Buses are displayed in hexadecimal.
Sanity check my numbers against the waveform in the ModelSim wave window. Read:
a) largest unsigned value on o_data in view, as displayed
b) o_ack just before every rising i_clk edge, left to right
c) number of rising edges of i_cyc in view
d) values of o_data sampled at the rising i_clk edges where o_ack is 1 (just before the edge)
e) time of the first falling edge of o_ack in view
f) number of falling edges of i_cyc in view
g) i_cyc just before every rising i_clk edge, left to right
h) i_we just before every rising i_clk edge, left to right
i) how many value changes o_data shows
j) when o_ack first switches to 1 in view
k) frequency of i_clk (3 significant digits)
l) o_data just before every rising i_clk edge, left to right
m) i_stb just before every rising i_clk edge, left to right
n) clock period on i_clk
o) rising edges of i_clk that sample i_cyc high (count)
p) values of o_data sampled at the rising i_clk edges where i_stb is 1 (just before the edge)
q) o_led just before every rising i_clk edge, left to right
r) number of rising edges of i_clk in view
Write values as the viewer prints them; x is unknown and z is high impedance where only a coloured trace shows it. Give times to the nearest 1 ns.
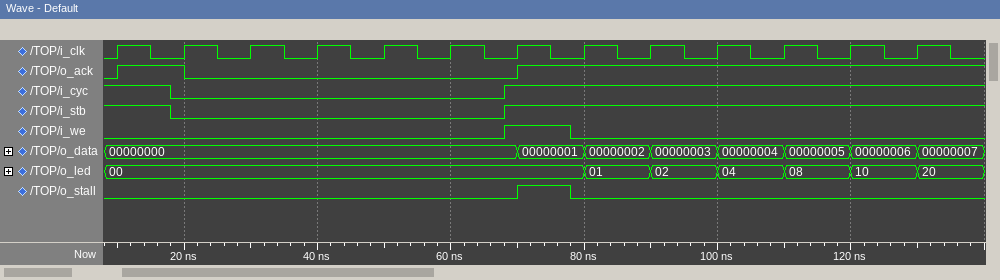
00000007
0 1 0 0 0 0 0 1 1 1 1 1 1
1
00000000, 00000001, 00000002, 00000003, 00000004, 00000005, 00000006
20 ns
1
1 0 0 0 0 0 1 1 1 1 1 1 1
0 0 0 0 0 0 1 0 0 0 0 0 0
7
10 ns
100 MHz
00000000, 00000000, 00000000, 00000000, 00000000, 00000000, 00000000, 00000001, 00000002, 00000003, 00000004, 00000005, 00000006
1 0 0 0 0 0 1 1 1 1 1 1 1
10 ns
8
00000000, 00000000, 00000001, 00000002, 00000003, 00000004, 00000005, 00000006
00, 00, 00, 00, 00, 00, 00, 00, 01, 02, 04, 08, 10
13
